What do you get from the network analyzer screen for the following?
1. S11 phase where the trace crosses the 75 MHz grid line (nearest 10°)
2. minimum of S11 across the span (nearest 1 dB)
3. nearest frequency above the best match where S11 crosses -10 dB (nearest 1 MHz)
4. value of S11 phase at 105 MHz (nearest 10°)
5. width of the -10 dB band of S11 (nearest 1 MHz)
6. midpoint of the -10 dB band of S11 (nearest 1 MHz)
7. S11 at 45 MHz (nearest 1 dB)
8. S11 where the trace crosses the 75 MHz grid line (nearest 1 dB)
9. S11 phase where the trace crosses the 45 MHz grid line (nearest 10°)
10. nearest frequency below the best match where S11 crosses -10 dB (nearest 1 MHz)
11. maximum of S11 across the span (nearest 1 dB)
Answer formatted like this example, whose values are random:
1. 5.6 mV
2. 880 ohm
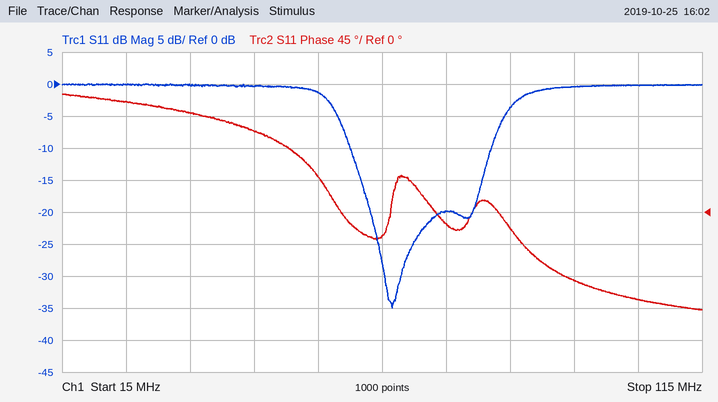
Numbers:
1. -20°
2. -35 dB
3. 82 MHz
4. -120°
5. 22 MHz
6. 71 MHz
7. 0 dB
8. -20 dB
9. 110°
10. 60 MHz
11. 0 dB
